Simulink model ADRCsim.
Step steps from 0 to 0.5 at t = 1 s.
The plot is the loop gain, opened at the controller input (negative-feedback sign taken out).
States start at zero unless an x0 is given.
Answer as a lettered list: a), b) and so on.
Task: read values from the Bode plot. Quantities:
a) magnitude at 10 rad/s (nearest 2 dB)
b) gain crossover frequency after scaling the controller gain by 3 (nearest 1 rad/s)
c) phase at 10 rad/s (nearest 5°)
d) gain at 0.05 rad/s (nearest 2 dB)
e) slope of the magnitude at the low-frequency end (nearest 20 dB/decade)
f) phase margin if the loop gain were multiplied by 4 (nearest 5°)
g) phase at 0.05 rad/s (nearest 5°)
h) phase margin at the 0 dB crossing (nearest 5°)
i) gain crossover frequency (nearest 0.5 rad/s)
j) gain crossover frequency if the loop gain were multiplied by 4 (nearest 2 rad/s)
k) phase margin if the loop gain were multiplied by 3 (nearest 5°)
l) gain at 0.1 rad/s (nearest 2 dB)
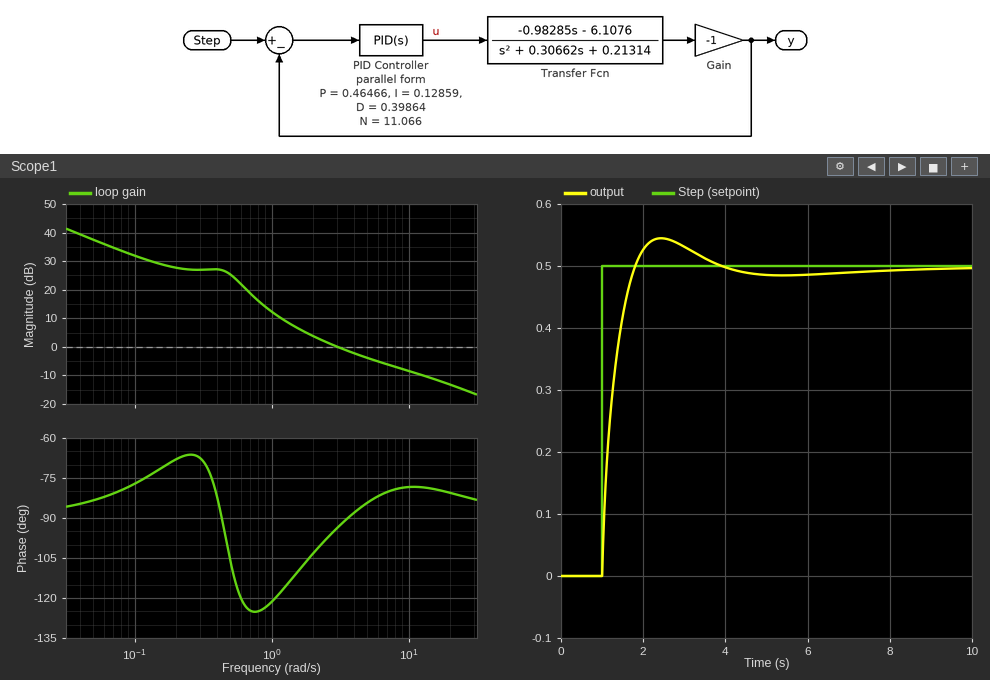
a) -8 dB
b) 12 rad/s
c) -80°
d) 38 dB
e) -20 dB/decade
f) 100°
g) -85°
h) 85°
i) 3.0 rad/s
j) 18 rad/s
k) 100°
l) 32 dB
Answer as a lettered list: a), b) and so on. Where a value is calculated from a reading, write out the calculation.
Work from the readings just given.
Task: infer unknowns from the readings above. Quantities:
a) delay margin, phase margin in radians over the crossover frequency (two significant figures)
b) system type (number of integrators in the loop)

a) 85 × π / 180 / 3 = 0.49 s
b) 1
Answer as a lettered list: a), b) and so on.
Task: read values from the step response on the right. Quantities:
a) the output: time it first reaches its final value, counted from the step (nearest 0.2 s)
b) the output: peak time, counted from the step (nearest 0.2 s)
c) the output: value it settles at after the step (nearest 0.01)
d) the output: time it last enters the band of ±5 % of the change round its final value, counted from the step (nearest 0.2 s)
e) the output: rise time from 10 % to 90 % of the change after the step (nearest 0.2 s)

a) 0.8 s
b) 1.4 s
c) 0.50
d) 2.2 s
e) 0.6 s
